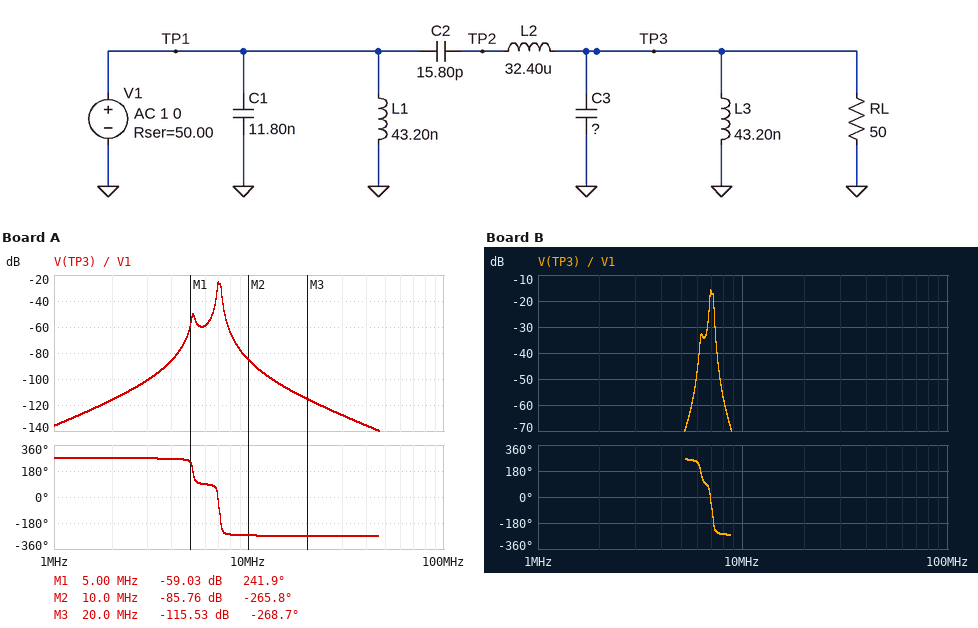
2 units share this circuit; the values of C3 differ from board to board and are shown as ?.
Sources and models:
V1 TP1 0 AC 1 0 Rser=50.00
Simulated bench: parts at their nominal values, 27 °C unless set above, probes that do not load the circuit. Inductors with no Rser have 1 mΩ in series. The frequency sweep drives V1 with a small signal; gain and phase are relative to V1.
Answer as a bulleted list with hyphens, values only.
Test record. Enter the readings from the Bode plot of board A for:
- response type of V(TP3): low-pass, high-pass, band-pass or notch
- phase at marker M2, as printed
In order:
- band-pass
- -265.8 deg
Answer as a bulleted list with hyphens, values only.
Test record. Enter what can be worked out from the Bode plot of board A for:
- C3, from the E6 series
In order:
- 22 nF
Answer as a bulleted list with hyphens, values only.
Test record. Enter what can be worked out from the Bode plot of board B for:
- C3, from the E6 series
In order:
- 15 nF
